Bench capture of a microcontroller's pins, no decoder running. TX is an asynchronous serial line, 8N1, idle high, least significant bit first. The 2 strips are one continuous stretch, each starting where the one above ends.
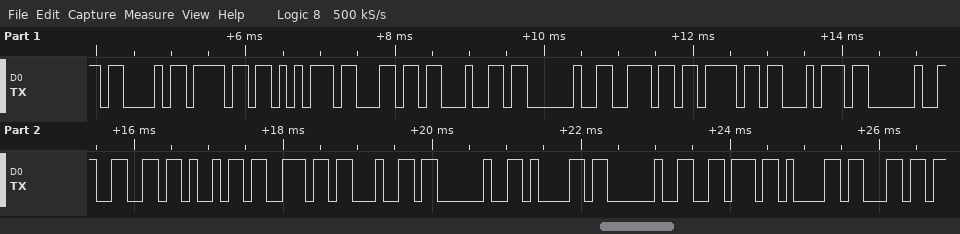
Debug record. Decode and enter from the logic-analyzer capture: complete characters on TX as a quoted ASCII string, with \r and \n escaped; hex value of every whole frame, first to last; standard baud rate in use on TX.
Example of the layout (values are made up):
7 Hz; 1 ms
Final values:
"Could not find a val"; 43 6F 75 6C 64 20 6E 6F 74 20 66 69 6E 64 20 61 20 76 61 6C; 9600 baud
